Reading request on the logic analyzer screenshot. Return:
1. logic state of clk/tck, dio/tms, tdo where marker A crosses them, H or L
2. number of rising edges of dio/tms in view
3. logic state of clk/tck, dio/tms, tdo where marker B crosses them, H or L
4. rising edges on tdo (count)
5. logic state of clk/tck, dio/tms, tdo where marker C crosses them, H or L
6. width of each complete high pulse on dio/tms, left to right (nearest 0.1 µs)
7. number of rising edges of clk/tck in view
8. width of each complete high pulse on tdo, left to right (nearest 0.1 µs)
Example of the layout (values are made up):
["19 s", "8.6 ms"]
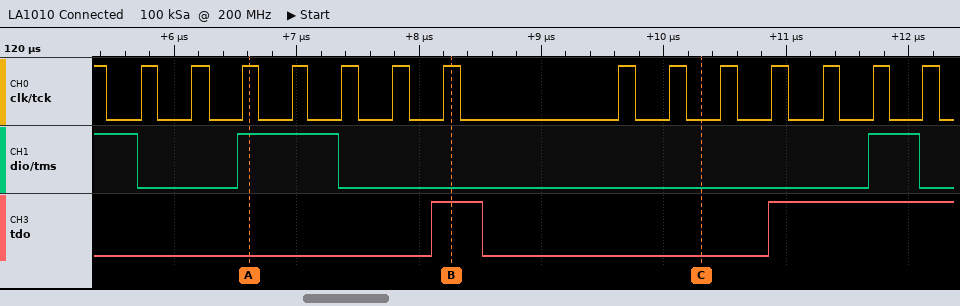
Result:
["clk/tck=H, dio/tms=H, tdo=L", "2", "clk/tck=H, dio/tms=L, tdo=H", "2", "clk/tck=L, dio/tms=L, tdo=L", "0.8 µs, 0.4 µs", "14", "0.4 µs"]
